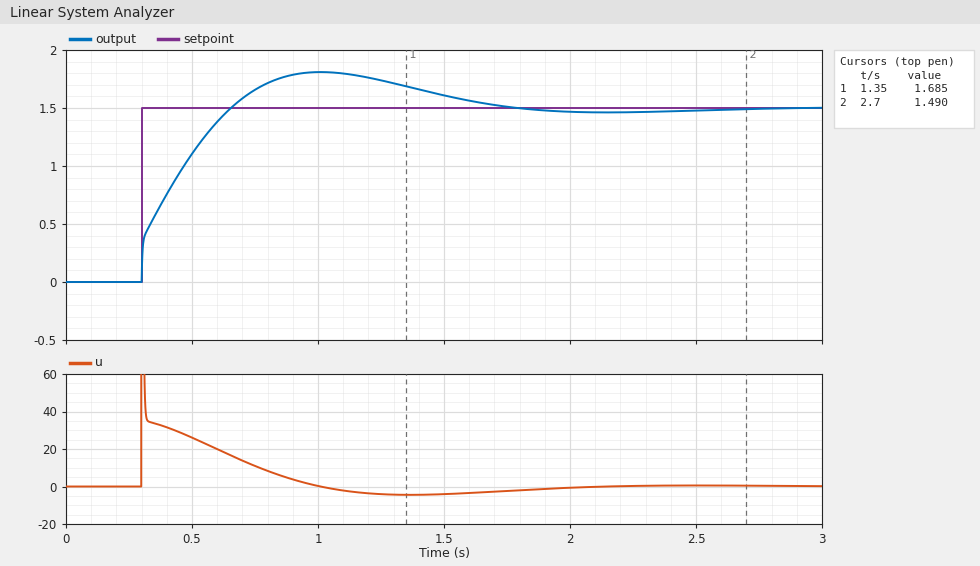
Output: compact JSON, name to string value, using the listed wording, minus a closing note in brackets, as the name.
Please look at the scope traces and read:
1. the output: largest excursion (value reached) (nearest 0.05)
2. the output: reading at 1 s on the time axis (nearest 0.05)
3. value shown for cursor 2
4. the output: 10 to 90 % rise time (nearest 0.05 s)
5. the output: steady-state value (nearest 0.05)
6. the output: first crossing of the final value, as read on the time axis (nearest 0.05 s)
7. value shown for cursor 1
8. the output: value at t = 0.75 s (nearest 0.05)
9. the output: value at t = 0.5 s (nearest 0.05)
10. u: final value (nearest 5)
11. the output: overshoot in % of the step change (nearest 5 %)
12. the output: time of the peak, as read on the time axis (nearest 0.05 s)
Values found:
{"the output: largest excursion (value reached)": "1.80", "the output: reading at 1 s on the time axis": "1.80", "value shown for cursor 2": "1.490", "the output: 10 to 90 % rise time": "0.30 s", "the output: steady-state value": "1.50", "the output: first crossing of the final value, as read on the time axis": "0.65 s", "value shown for cursor 1": "1.685", "the output: value at t = 0.75 s": "1.65", "the output: value at t = 0.5 s": "1.10", "u: final value": "0", "the output: overshoot in % of the step change": "20 %", "the output: time of the peak, as read on the time axis": "1.00 s"}
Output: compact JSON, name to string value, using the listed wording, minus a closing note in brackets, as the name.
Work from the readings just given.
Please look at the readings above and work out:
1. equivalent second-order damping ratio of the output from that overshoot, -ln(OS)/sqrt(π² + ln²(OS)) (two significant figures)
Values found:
{"equivalent second-order damping ratio of the output from that overshoot, -ln(OS)/sqrt(π² + ln²(OS))": "0.46"}
